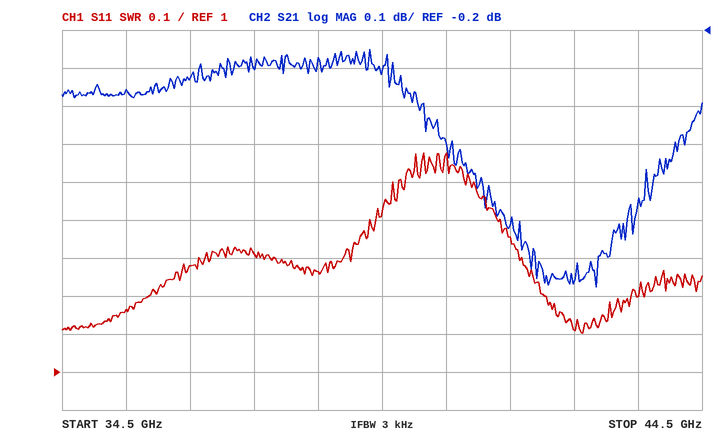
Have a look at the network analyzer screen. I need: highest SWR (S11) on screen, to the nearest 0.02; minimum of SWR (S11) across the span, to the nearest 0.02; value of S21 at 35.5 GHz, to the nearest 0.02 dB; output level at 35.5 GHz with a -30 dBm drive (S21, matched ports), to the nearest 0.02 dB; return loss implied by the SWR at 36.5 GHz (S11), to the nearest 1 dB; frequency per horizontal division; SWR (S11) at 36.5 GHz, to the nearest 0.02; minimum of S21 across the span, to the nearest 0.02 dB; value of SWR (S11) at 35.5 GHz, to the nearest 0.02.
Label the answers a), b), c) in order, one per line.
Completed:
a) 1.58
b) 1.10
c) -0.36 dB
d) -30.36 dBm
e) 18 dB
f) 1 GHz
g) 1.28
h) -0.88 dB
i) 1.16
